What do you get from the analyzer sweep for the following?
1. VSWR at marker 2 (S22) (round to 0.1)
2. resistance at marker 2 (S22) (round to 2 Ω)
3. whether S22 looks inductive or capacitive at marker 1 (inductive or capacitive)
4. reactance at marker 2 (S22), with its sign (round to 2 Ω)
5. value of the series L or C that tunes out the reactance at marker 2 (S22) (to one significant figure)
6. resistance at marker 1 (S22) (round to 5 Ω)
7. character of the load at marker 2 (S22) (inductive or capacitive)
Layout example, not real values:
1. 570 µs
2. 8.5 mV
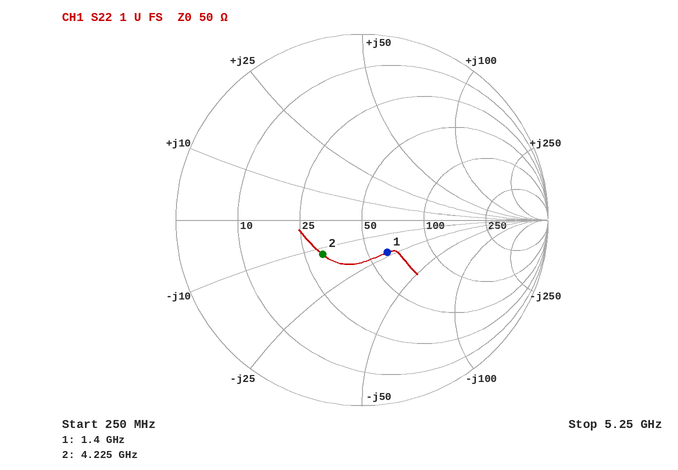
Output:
1. 1.8
2. 30 Ω
3. capacitive
4. -12 Ω
5. 500 pH
6. 60 Ω
7. capacitive
